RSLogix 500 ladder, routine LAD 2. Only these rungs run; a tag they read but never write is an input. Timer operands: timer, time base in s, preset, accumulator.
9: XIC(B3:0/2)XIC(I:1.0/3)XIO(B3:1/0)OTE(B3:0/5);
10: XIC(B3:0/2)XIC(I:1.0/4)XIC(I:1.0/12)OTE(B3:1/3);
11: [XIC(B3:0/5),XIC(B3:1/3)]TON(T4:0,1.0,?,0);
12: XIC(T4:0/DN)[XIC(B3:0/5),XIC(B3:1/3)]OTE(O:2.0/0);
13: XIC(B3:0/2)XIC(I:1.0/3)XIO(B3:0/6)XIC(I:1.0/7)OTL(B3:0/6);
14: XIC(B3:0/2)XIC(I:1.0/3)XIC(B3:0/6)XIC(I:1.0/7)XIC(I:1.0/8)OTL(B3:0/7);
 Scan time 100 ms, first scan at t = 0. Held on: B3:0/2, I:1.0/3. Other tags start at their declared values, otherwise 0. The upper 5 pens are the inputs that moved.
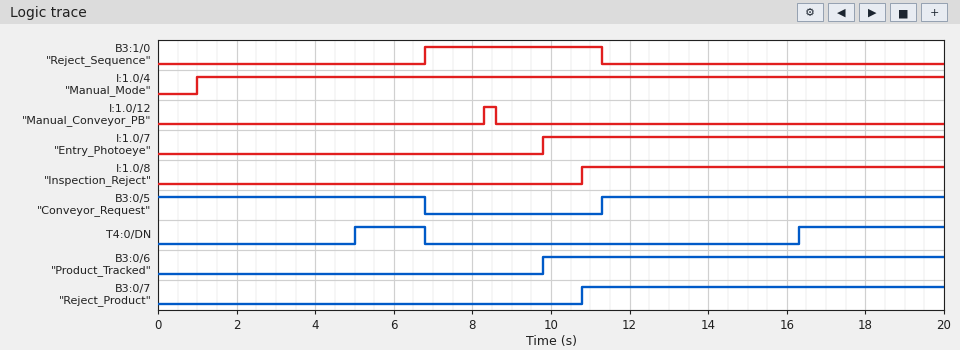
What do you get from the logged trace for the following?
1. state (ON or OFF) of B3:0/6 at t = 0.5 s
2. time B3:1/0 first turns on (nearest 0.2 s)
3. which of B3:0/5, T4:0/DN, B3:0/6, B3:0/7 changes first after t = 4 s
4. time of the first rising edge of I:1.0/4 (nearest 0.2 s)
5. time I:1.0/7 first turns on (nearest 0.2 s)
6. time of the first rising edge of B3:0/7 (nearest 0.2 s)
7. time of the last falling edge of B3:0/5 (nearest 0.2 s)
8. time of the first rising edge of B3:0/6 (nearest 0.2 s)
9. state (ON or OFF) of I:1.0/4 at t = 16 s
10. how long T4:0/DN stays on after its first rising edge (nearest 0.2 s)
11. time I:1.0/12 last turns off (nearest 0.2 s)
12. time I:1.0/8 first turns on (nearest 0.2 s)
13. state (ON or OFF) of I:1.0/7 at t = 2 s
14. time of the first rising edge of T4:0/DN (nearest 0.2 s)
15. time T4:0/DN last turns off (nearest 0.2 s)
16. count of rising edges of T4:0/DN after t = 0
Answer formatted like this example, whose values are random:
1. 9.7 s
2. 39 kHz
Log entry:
1. OFF
2. 6.8 s
3. T4:0/DN
4. 1.0 s
5. 9.8 s
6. 10.8 s
7. 6.8 s
8. 9.8 s
9. ON
10. 1.8 s
11. 8.6 s
12. 10.8 s
13. OFF
14. 5.0 s
15. 6.8 s
16. 2
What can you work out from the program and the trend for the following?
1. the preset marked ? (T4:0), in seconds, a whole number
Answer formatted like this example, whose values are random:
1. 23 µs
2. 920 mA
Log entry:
1. 5 s
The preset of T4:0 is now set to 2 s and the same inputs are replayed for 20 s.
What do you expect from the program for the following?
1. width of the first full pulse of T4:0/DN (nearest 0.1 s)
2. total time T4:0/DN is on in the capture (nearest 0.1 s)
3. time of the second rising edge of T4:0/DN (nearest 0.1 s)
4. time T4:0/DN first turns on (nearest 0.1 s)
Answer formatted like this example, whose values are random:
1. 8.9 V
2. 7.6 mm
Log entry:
1. 4.8 s
2. 11.5 s
3. 13.3 s
4. 2.0 s
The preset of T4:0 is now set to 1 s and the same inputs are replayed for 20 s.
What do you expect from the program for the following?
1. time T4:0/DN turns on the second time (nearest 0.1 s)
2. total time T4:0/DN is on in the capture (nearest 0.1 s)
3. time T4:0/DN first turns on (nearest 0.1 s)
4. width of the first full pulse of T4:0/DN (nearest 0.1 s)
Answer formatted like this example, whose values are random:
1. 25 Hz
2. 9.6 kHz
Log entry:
1. 12.3 s
2. 13.5 s
3. 1.0 s
4. 5.8 s
